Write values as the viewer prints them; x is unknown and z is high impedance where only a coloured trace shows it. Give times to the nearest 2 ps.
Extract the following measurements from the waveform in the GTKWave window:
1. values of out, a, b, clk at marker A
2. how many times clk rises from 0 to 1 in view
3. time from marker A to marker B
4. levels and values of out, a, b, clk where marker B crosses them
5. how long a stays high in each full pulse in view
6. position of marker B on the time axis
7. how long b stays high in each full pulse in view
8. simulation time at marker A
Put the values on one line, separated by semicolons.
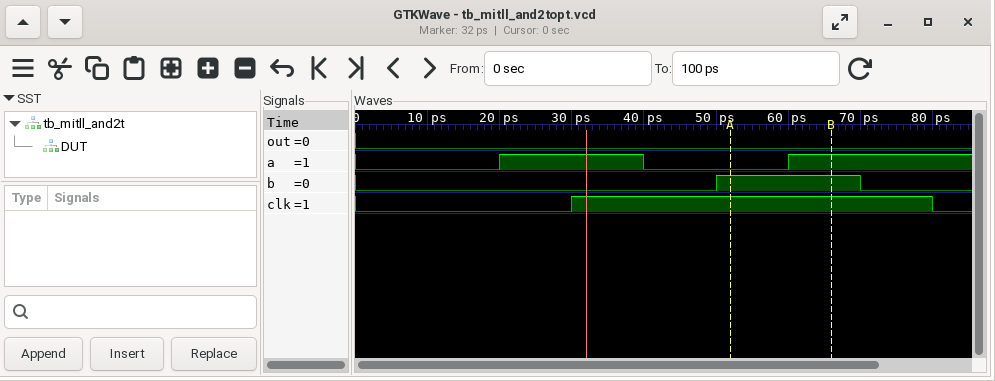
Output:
out=0, a=0, b=1, clk=1; 1; 14 ps; out=0, a=1, b=1, clk=1; 20 ps; 66 ps; 20 ps; 52 ps
